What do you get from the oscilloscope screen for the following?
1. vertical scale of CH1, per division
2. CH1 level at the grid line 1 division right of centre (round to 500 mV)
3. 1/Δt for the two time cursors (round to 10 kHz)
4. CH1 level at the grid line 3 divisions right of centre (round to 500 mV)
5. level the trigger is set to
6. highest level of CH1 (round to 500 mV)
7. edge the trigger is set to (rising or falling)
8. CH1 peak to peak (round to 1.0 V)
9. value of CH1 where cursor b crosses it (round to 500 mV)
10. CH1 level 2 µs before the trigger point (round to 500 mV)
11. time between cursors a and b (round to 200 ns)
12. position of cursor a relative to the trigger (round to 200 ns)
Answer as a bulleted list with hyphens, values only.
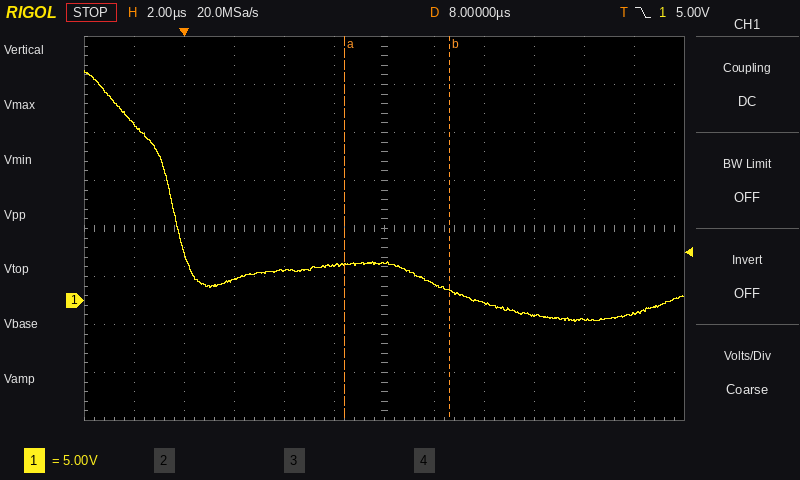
- 5 V
- 1.5 V
- 240 kHz
- -1.5 V
- 5.00 V
- 24.0 V
- falling
- 26.0 V
- 1.0 V
- 18.5 V
- 4.2 µs
- +6.4 µs
